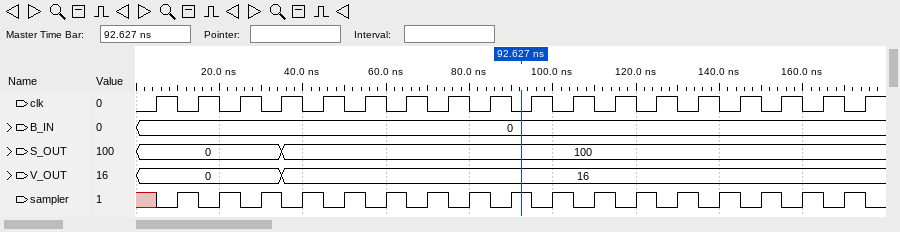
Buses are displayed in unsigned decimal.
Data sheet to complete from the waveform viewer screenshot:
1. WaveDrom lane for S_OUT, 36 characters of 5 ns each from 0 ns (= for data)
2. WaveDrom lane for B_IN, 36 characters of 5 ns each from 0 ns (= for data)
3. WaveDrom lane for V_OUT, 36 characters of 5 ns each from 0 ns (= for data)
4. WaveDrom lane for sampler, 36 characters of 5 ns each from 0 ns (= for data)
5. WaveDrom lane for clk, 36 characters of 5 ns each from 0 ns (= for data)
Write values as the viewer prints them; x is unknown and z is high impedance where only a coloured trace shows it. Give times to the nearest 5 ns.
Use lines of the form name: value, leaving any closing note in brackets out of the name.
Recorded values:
WaveDrom lane for S_OUT, 36 characters of 5 ns each from 0 ns: {name: 'S_OUT', wave: '=......=............................', data: '0 100'}
WaveDrom lane for B_IN, 36 characters of 5 ns each from 0 ns: {name: 'B_IN', wave: '=...................................', data: '0'}
WaveDrom lane for V_OUT, 36 characters of 5 ns each from 0 ns: {name: 'V_OUT', wave: '=......=............................', data: '0 16'}
WaveDrom lane for sampler, 36 characters of 5 ns each from 0 ns: {name: 'sampler', wave: 'x01010101010101010101010101010101010'}
WaveDrom lane for clk, 36 characters of 5 ns each from 0 ns: {name: 'clk', wave: '010101010101010101010101010101010101'}
